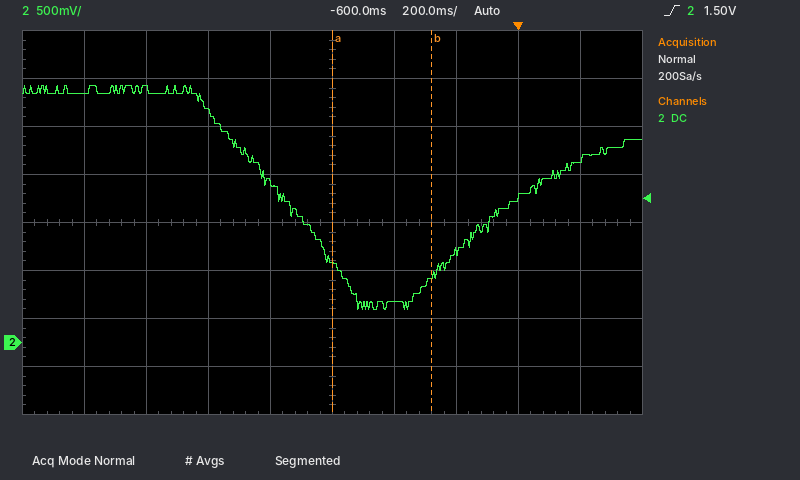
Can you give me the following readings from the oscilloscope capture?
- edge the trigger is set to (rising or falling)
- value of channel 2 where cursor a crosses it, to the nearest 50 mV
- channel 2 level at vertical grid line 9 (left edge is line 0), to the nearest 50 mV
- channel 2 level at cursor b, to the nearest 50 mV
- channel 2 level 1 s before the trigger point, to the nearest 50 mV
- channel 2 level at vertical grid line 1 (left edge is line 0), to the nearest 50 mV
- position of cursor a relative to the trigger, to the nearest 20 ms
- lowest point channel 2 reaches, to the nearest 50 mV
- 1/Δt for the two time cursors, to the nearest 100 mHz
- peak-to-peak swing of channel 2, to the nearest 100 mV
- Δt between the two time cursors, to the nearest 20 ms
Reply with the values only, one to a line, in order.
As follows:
rising
850 mV
1.90 V
700 mV
2.40 V
2.60 V
-600 ms
350 mV
3.1 Hz
2.30 V
320 ms
